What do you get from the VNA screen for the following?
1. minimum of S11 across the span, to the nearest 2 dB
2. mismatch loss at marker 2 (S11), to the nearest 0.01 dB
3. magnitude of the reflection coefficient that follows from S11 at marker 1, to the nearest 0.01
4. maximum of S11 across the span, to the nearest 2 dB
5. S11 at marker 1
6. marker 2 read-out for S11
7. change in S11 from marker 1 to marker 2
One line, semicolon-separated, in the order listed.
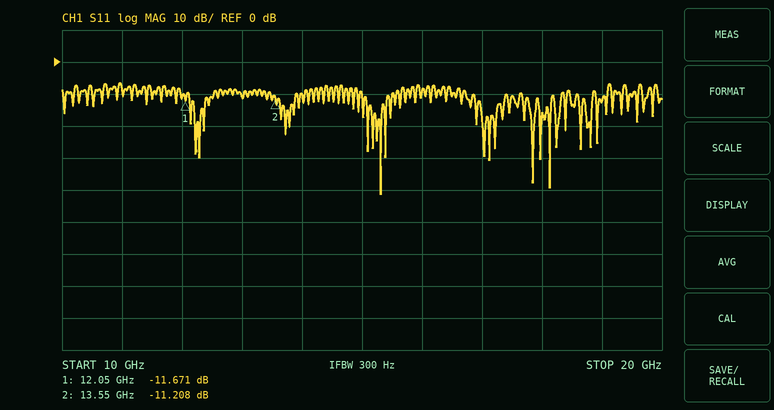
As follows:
-42 dB; 0.34 dB; 0.26; -6 dB; -11.671 dB; -11.208 dB; 0.463 dB
